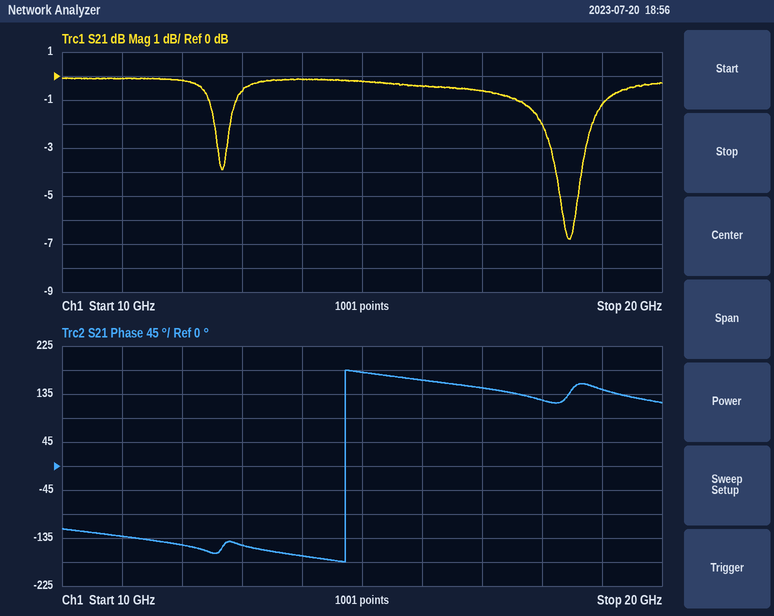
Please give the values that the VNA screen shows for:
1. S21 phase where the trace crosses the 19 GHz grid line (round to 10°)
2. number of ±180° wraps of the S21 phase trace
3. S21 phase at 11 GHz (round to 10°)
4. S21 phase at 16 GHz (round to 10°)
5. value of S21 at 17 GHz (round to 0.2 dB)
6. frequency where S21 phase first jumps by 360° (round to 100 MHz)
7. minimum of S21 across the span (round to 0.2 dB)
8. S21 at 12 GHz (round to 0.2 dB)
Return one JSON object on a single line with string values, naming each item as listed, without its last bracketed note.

{"S21 phase where the trace crosses the 19 GHz grid line": "140°", "number of ±180° wraps of the S21 phase trace": "1", "S21 phase at 11 GHz": "-130°", "S21 phase at 16 GHz": "160°", "value of S21 at 17 GHz": "-0.6 dB", "frequency where S21 phase first jumps by 360°": "14.7 GHz", "minimum of S21 across the span": "-6.8 dB", "S21 at 12 GHz": "-0.2 dB"}
